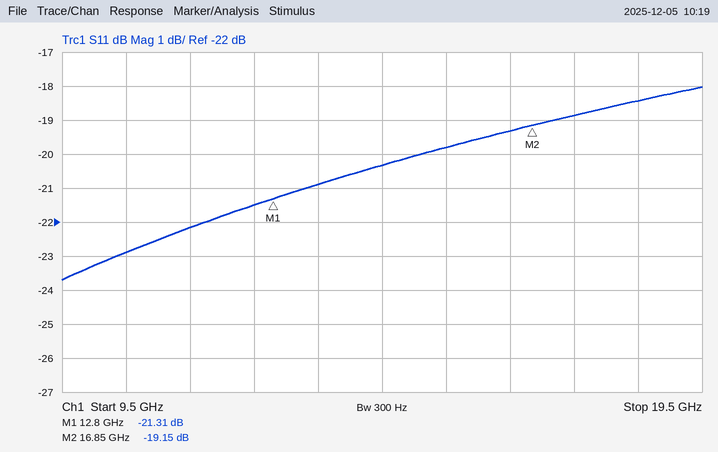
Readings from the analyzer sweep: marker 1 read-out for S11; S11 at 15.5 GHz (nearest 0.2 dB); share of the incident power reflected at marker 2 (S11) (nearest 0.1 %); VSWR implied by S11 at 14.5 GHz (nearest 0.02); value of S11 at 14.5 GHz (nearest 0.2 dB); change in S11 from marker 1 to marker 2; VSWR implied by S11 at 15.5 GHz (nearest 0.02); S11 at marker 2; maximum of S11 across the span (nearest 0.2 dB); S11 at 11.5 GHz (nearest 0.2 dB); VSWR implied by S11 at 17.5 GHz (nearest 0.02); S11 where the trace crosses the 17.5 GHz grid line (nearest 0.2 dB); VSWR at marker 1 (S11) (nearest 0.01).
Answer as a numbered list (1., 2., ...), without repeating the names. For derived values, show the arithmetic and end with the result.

1. -21.31 dB
2. -19.8 dB
3. 10^(-19.15/10) ≈ 1.2 %
4. |Γ| = 10^(-20.4/20) = 0.0955; VSWR = (1 + 0.0955)/(1 − 0.0955) ≈ 1.21, so 1.22 to the nearest 0.02
5. -20.4 dB
6. -19.15 − (-21.31) = 2.16 dB
7. |Γ| = 10^(-19.8/20) = 0.1023; VSWR = (1 + 0.1023)/(1 − 0.1023) ≈ 1.23, so 1.22 to the nearest 0.02
8. -19.15 dB
9. -18.0 dB
10. -22.2 dB
11. |Γ| = 10^(-18.8/20) = 0.1148; VSWR = (1 + 0.1148)/(1 − 0.1148) ≈ 1.26
12. -18.8 dB
13. (1 + 0.0860)/(1 − 0.0860) ≈ 1.19
